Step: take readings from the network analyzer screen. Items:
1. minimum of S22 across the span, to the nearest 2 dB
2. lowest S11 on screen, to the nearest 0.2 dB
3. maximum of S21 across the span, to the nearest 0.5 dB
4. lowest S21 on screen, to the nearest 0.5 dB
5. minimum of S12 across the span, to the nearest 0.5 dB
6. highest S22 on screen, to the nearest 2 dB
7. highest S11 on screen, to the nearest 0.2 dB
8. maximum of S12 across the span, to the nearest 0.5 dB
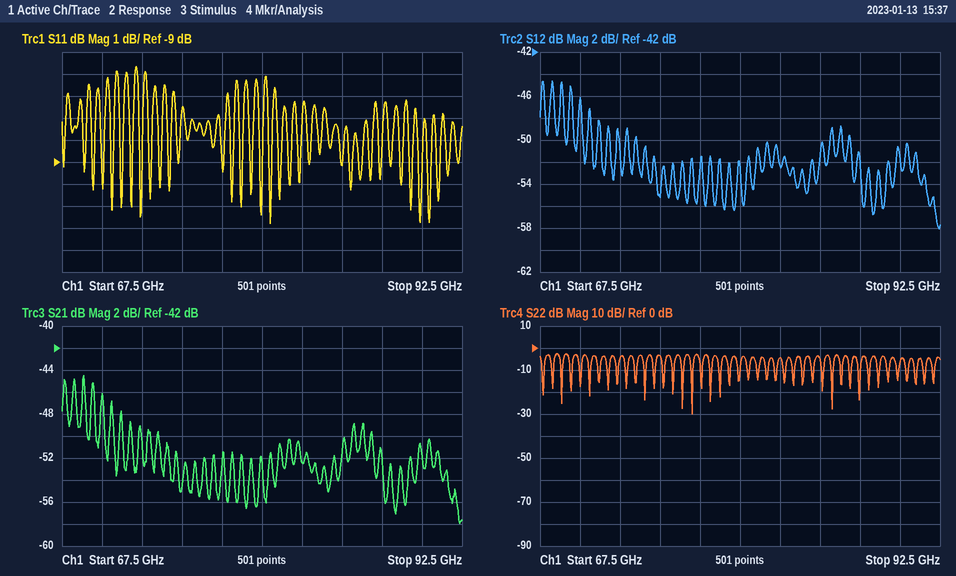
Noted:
-30 dB
-11.8 dB
-44.5 dB
-58.0 dB
-58.0 dB
-2 dB
-4.6 dB
-44.5 dB
